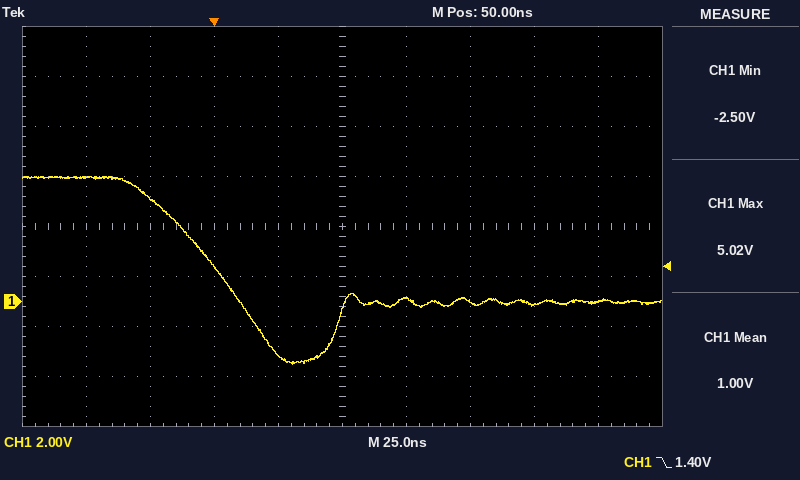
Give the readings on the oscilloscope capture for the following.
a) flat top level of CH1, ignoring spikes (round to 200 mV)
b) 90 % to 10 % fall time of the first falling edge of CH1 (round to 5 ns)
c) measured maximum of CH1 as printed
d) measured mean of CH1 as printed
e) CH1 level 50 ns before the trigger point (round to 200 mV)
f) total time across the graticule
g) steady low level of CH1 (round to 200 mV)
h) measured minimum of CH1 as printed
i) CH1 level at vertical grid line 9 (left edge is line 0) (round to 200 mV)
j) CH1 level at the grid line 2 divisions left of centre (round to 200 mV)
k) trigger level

5.0 V
35 ns
5.02 V
1.00 V
5.0 V
250 ns
0.0 V
-2.50 V
0.0 V
1.4 V
1.40 V
